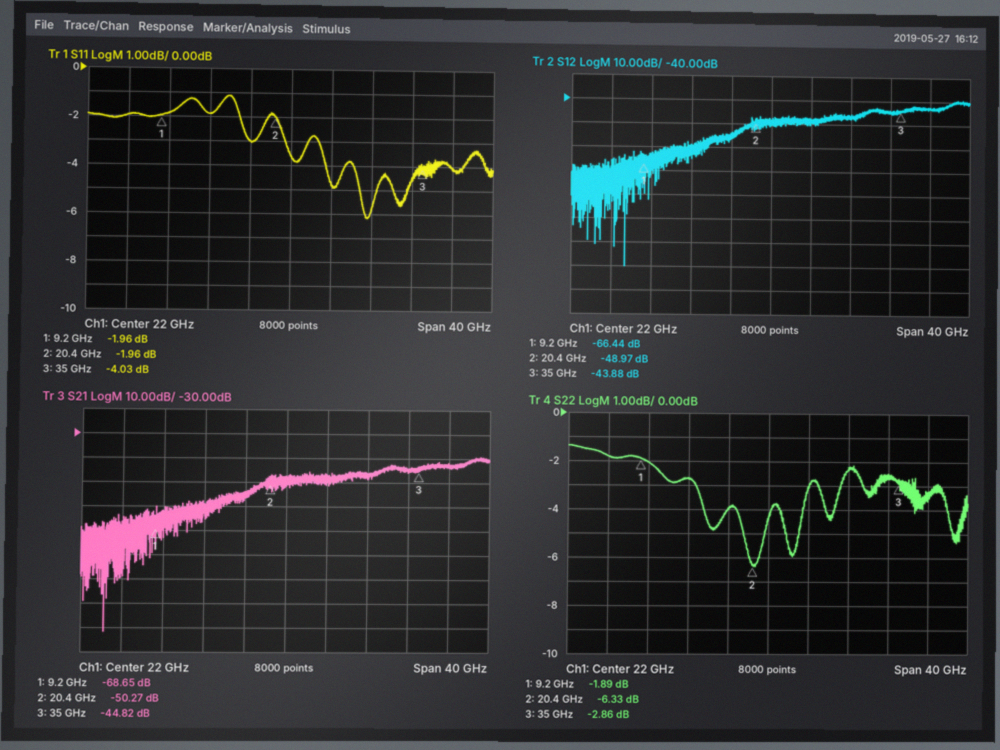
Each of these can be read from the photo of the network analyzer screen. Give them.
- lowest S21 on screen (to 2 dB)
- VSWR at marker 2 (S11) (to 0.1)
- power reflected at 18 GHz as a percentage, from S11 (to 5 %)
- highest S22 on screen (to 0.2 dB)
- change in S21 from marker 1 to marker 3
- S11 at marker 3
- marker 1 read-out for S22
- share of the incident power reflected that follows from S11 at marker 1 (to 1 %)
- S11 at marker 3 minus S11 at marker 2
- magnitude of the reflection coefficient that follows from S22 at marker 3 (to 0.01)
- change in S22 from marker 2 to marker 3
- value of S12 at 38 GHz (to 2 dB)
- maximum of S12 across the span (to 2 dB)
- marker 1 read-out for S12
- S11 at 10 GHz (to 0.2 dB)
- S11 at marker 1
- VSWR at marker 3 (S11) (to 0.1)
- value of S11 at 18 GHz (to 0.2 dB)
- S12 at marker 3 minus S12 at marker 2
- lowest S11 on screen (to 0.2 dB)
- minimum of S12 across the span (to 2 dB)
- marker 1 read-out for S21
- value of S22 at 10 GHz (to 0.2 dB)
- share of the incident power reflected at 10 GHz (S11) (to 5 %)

-112 dB
8.9
50 %
-1.4 dB
23.83 dB
-4.03 dB
-1.89 dB
64 %
-2.07 dB
0.72
3.47 dB
-44 dB
-40 dB
-66.44 dB
-1.8 dB
-1.96 dB
4.4
-3.0 dB
5.09 dB
-6.2 dB
-110 dB
-68.65 dB
-2.0 dB
65 %
